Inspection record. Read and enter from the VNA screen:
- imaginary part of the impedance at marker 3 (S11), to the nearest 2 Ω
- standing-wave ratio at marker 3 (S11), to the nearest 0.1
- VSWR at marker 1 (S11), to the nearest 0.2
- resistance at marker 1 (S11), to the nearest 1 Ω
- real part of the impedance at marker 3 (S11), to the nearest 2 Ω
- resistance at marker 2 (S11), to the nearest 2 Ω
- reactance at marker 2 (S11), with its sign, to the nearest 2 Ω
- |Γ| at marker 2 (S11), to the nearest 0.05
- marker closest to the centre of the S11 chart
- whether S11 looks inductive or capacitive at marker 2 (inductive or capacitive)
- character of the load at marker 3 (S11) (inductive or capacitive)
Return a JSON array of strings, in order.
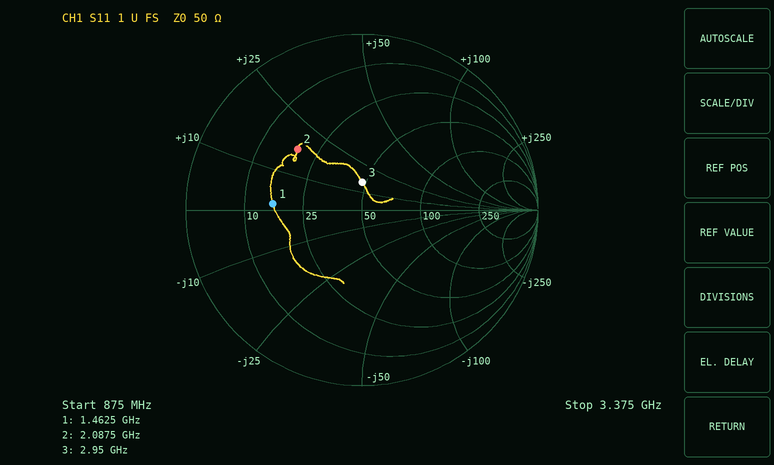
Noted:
["+16 Ω", "1.4", "3.0", "16 Ω", "48 Ω", "18 Ω", "+18 Ω", "0.50", "marker 3", "inductive", "inductive"]
